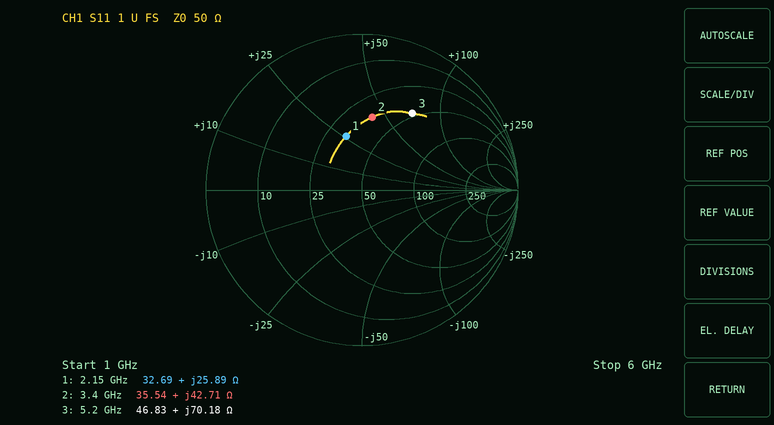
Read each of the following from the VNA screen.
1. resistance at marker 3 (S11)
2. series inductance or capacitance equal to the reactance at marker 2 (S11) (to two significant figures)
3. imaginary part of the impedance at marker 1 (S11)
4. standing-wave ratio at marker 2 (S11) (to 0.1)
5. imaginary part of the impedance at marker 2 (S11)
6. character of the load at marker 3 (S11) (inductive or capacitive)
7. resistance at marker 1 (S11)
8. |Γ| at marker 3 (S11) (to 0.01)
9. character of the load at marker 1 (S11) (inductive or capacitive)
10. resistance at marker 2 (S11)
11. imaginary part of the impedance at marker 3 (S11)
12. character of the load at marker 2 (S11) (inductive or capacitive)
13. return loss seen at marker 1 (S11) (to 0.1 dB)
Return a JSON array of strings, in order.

["46.83 Ω", "2.0 nH", "+25.89 Ω", "2.8", "+42.71 Ω", "inductive", "32.69 Ω", "0.59", "inductive", "35.54 Ω", "+70.18 Ω", "inductive", "8.9 dB"]
